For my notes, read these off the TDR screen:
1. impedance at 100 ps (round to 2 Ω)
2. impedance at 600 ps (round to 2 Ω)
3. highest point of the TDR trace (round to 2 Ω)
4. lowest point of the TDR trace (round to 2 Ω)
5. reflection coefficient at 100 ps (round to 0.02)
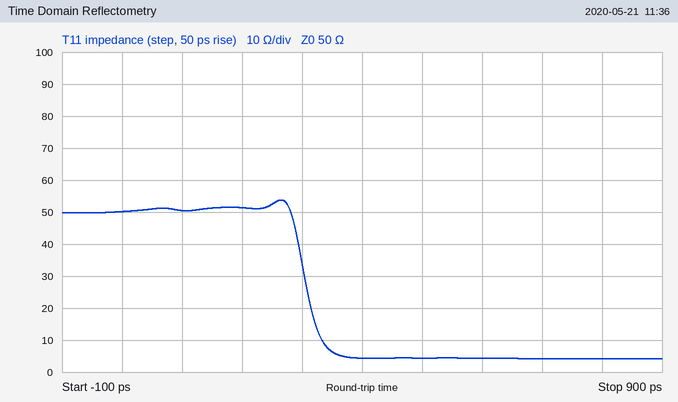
50 Ω
4 Ω
54 Ω
4 Ω
0.00
